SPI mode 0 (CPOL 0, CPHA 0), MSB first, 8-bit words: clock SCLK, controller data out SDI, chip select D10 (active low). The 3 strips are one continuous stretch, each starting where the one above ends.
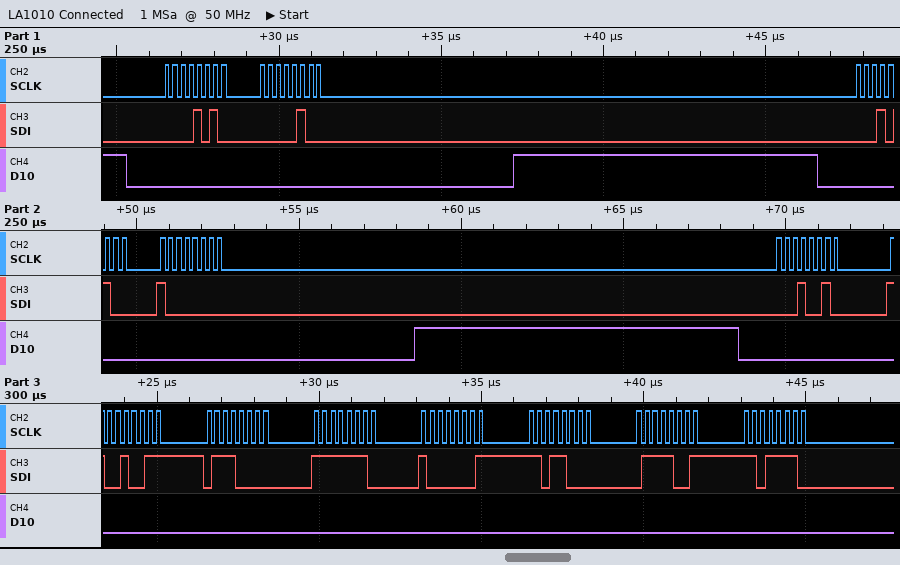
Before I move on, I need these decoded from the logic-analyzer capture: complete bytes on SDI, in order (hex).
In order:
0A 04 14 80 12 93 70 FE 81 D8 79 DE
